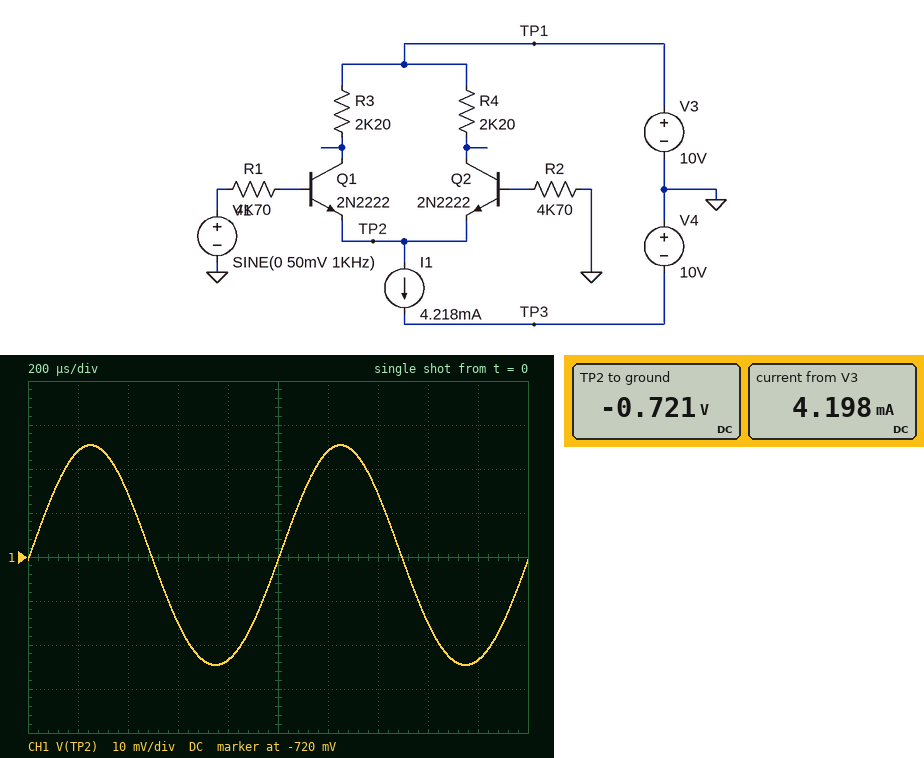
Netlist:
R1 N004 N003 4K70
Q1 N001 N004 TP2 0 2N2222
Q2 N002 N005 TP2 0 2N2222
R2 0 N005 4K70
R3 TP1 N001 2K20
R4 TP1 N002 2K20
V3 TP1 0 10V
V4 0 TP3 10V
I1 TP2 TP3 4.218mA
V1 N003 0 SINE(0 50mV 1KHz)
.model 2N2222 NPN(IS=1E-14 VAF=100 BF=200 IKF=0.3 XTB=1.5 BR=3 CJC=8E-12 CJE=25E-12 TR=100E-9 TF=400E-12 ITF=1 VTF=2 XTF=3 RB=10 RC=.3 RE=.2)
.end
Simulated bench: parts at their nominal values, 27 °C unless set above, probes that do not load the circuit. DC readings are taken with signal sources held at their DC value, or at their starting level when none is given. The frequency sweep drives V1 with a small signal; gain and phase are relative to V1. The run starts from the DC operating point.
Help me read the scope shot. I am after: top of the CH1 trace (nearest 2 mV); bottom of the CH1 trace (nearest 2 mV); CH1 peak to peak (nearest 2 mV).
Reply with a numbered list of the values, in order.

1. -694 mV
2. -744 mV
3. 50 mV
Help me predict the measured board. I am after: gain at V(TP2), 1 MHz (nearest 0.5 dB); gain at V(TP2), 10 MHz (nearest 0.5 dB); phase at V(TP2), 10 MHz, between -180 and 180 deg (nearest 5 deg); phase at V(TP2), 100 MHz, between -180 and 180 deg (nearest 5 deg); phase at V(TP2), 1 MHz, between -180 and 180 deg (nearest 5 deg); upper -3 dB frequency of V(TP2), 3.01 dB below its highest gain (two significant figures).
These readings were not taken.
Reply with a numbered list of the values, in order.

1. -6.0 dB
2. -11.0 dB
3. -30 deg
4. -5 deg
5. -5 deg
6. 6.5 MHz
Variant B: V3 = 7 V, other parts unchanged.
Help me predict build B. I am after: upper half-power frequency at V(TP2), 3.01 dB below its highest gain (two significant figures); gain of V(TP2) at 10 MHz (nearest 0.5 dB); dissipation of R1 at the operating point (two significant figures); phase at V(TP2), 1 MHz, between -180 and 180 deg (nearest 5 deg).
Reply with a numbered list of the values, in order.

1. 5.2 MHz
2. -12.0 dB
3. 500 nW
4. -10 deg
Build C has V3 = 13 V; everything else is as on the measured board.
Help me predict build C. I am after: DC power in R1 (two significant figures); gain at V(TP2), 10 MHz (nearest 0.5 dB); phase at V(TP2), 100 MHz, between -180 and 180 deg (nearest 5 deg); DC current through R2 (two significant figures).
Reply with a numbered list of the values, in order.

1. 450 nW
2. -10.5 dB
3. -10 deg
4. 9.7 µA
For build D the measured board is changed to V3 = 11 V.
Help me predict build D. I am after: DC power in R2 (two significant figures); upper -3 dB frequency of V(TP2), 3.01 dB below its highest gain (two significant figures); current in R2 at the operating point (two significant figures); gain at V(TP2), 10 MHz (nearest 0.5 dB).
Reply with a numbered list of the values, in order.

1. 460 nW
2. 6.8 MHz
3. 9.9 µA
4. -10.5 dB
